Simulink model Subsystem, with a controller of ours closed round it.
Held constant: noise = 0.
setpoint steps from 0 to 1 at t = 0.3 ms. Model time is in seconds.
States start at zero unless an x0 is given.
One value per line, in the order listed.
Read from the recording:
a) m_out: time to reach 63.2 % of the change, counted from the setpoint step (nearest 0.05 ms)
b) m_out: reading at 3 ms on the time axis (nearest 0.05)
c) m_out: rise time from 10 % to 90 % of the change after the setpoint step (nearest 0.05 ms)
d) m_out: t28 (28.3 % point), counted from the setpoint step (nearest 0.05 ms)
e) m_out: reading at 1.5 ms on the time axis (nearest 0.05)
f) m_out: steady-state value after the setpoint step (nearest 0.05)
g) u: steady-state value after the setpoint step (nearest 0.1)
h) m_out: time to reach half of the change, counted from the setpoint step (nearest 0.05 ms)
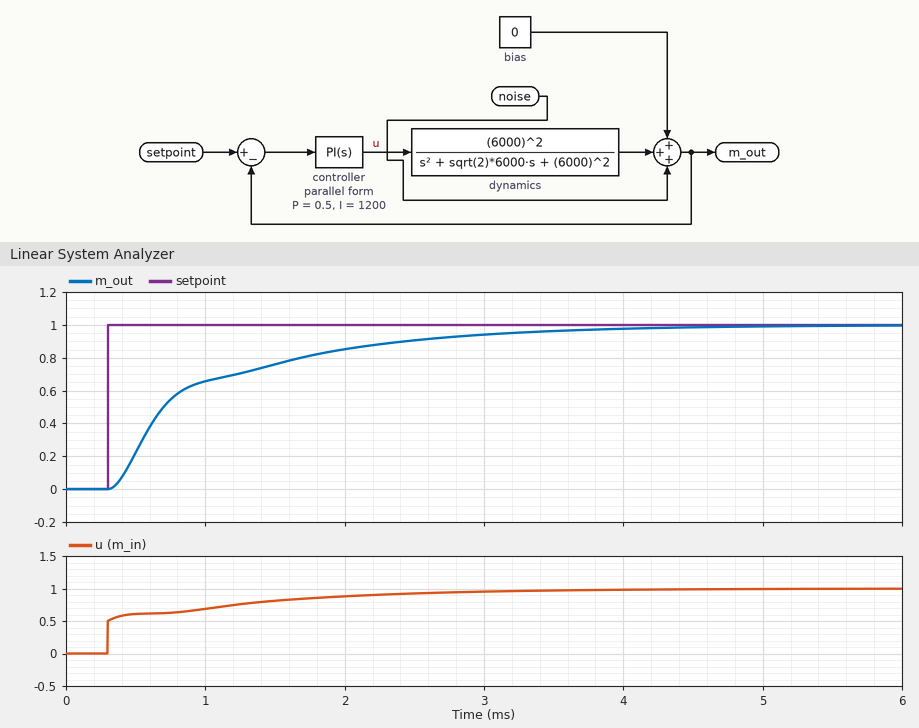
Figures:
0.60 ms
0.95
2.00 ms
0.25 ms
0.75
1.00
1.0
0.40 ms
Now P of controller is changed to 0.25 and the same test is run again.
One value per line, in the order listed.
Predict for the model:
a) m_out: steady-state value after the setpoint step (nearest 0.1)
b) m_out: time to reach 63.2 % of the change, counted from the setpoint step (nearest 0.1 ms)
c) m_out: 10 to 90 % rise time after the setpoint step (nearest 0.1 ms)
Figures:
1.0
0.8 ms
1.7 ms
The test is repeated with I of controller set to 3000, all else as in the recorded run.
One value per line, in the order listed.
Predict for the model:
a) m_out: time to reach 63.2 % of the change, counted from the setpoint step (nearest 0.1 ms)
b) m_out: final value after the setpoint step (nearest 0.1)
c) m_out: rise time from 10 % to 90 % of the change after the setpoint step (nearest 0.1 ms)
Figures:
0.4 ms
1.0
0.4 ms
